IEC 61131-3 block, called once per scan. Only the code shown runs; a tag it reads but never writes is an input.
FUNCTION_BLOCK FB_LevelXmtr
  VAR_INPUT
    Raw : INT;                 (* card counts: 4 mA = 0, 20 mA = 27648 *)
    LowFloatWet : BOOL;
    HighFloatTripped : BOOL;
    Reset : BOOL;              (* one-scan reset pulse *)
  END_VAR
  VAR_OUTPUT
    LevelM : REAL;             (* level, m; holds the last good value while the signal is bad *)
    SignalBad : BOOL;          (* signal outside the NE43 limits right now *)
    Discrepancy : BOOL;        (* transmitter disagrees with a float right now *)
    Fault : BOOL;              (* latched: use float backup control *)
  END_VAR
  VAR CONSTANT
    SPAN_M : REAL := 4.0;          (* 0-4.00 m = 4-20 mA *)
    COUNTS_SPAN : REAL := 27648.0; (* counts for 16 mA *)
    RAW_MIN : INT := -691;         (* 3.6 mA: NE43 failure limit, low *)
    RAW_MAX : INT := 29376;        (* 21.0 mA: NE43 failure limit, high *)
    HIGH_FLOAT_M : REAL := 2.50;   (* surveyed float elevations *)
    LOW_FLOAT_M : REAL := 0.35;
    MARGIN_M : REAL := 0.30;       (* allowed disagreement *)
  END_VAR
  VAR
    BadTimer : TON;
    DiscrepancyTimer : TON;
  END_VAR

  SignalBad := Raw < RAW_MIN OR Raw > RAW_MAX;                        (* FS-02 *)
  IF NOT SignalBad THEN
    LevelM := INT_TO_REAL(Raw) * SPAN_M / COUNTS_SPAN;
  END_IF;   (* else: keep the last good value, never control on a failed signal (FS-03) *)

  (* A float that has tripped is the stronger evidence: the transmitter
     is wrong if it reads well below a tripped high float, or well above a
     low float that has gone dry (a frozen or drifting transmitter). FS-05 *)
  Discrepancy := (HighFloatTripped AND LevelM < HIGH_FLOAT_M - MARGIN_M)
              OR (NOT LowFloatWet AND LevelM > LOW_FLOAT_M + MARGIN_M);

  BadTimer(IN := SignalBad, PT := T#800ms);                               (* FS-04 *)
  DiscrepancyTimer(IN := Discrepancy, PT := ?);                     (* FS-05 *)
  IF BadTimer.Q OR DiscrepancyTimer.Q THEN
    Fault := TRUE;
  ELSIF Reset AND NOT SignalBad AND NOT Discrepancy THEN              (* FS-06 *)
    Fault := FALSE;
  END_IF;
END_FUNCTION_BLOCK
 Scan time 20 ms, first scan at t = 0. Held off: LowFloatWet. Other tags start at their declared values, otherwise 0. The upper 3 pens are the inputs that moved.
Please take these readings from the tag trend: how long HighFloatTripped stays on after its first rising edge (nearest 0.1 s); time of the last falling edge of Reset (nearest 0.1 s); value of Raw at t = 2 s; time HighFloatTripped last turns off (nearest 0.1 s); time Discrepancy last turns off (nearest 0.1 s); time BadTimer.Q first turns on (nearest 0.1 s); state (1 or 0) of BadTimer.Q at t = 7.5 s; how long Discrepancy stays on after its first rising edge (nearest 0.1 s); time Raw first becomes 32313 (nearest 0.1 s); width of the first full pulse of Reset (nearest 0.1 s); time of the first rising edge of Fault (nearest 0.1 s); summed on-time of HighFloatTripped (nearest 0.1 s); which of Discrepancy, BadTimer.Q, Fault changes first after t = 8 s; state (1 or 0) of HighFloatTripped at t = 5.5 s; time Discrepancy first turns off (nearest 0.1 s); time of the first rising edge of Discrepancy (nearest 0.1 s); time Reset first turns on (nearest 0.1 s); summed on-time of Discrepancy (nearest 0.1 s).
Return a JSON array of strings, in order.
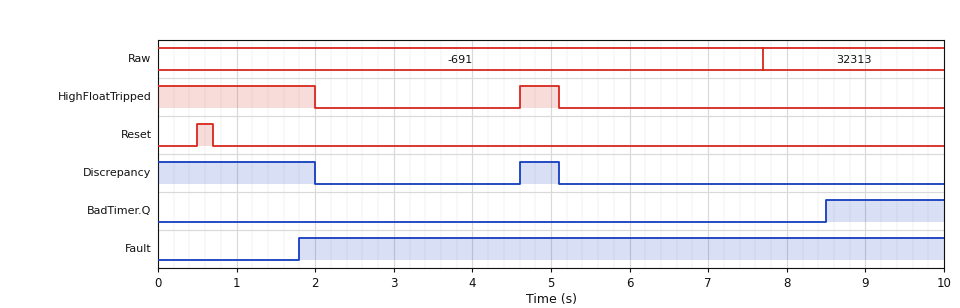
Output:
["0.5 s", "0.7 s", "-691", "5.1 s", "5.1 s", "8.5 s", "0", "0.5 s", "7.7 s", "0.2 s", "1.8 s", "2.5 s", "BadTimer.Q", "0", "2.0 s", "4.6 s", "0.5 s", "2.5 s"]
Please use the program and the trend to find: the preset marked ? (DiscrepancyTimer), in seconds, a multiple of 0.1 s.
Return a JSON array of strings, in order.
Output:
["1.8 s"]
